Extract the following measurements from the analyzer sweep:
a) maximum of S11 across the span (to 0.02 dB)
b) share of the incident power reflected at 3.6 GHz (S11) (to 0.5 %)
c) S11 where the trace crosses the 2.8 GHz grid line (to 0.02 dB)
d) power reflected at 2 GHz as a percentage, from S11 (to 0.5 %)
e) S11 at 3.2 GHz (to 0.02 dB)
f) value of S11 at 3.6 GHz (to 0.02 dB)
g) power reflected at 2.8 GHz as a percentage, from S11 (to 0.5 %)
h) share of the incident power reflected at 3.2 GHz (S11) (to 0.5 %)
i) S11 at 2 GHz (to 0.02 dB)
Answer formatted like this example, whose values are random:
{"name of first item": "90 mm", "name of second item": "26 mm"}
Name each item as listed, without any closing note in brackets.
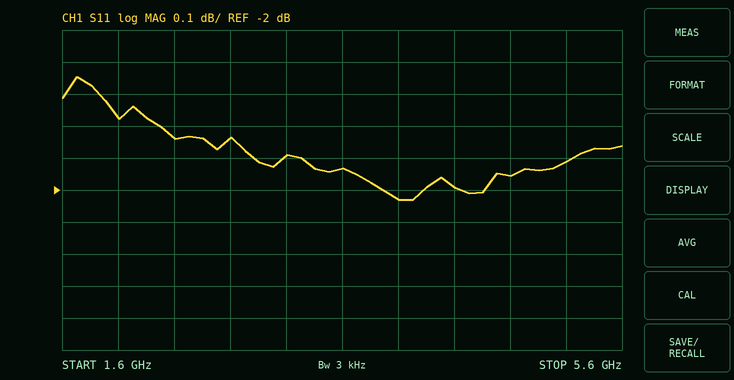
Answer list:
{"maximum of S11 across the span": "-1.64 dB", "share of the incident power reflected at 3.6 GHz (S11)": "64.0 %", "S11 where the trace crosses the 2.8 GHz grid line": "-1.84 dB", "power reflected at 2 GHz as a percentage, from S11": "66.5 %", "S11 at 3.2 GHz": "-1.90 dB", "value of S11 at 3.6 GHz": "-1.94 dB", "power reflected at 2.8 GHz as a percentage, from S11": "65.5 %", "share of the incident power reflected at 3.2 GHz (S11)": "64.5 %", "S11 at 2 GHz": "-1.78 dB"}
